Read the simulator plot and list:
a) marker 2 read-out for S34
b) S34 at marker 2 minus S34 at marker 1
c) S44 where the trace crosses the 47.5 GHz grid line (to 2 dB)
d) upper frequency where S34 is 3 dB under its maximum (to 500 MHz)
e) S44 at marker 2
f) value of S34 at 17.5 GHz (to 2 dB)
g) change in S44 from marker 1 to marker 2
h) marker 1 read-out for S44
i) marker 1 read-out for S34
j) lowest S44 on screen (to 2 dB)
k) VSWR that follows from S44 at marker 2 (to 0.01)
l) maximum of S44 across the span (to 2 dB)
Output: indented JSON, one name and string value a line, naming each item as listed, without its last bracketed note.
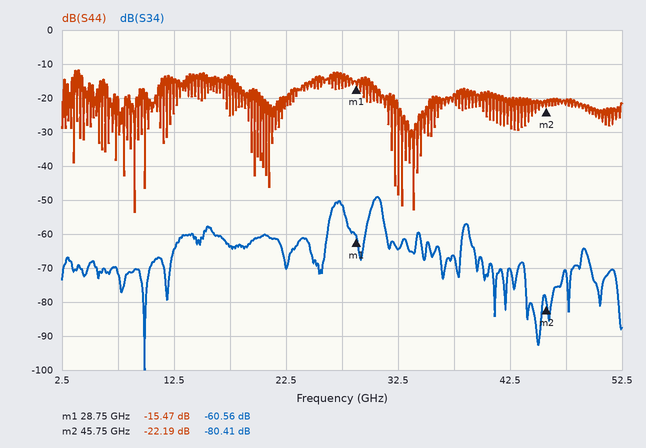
{
  "marker 2 read-out for S34": "-80.41 dB",
  "S34 at marker 2 minus S34 at marker 1": "-19.85 dB",
  "S44 where the trace crosses the 47.5 GHz grid line": "-22 dB",
  "upper frequency where S34 is 3 dB under its maximum": "31.0 GHz",
  "S44 at marker 2": "-22.19 dB",
  "value of S34 at 17.5 GHz": "-64 dB",
  "change in S44 from marker 1 to marker 2": "-6.72 dB",
  "marker 1 read-out for S44": "-15.47 dB",
  "marker 1 read-out for S34": "-60.56 dB",
  "lowest S44 on screen": "-54 dB",
  "VSWR that follows from S44 at marker 2": "1.17",
  "maximum of S44 across the span": "-12 dB"
}
